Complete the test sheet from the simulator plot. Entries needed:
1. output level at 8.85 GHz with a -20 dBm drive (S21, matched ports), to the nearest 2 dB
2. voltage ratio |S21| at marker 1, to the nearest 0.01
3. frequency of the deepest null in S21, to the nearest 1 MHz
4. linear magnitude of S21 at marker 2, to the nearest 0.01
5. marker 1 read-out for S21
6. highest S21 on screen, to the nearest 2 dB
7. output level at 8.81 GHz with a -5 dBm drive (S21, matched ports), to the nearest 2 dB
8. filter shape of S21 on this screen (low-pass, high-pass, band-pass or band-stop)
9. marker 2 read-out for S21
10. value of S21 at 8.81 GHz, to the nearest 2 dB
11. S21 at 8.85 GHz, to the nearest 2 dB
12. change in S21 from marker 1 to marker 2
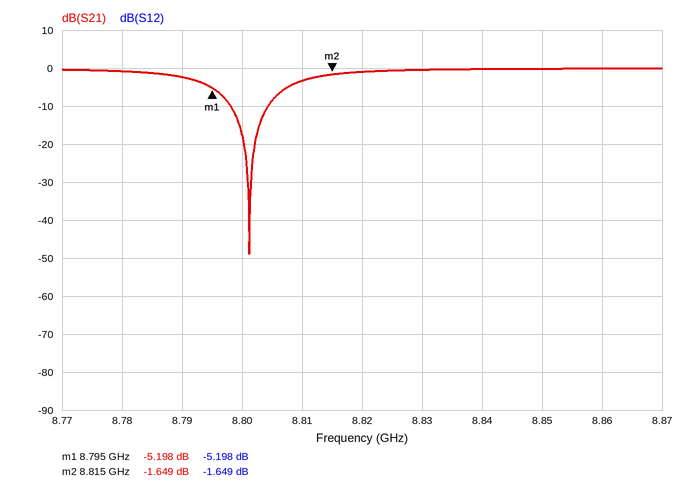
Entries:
-20 dBm
0.55
8.801 GHz
0.83
-5.198 dB
0 dB
-8 dBm
band-stop
-1.649 dB
-4 dB
0 dB
3.549 dB
